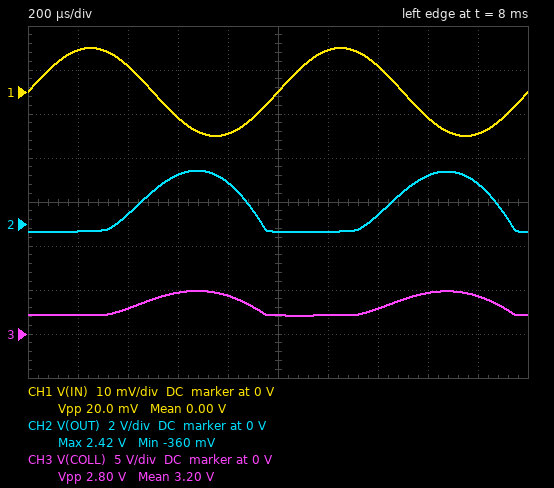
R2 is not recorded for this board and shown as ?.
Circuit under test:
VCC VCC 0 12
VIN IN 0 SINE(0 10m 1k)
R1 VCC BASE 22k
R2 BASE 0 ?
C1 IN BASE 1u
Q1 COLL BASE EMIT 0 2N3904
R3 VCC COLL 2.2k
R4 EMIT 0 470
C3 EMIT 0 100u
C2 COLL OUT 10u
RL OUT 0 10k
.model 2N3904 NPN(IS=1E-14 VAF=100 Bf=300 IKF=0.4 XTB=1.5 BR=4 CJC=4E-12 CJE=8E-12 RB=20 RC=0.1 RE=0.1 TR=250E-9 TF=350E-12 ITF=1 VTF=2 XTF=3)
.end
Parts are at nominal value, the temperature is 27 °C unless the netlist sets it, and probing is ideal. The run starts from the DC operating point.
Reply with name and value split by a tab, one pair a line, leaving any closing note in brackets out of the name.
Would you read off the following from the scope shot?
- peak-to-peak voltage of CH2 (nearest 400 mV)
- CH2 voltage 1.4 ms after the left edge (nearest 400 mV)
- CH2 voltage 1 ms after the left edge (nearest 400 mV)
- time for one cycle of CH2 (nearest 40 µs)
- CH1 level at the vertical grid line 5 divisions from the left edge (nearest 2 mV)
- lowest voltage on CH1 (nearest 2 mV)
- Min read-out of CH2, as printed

peak-to-peak voltage of CH2	2.8 V
CH2 voltage 1.4 ms after the left edge	400 mV
CH2 voltage 1 ms after the left edge	-400 mV
time for one cycle of CH2	1.00 ms
CH1 level at the vertical grid line 5 divisions from the left edge	0 V
lowest voltage on CH1	-10 mV
Min read-out of CH2, as printed	-360 mV
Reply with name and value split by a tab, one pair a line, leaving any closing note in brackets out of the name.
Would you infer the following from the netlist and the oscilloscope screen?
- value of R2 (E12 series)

value of R2	6.8 kΩ
